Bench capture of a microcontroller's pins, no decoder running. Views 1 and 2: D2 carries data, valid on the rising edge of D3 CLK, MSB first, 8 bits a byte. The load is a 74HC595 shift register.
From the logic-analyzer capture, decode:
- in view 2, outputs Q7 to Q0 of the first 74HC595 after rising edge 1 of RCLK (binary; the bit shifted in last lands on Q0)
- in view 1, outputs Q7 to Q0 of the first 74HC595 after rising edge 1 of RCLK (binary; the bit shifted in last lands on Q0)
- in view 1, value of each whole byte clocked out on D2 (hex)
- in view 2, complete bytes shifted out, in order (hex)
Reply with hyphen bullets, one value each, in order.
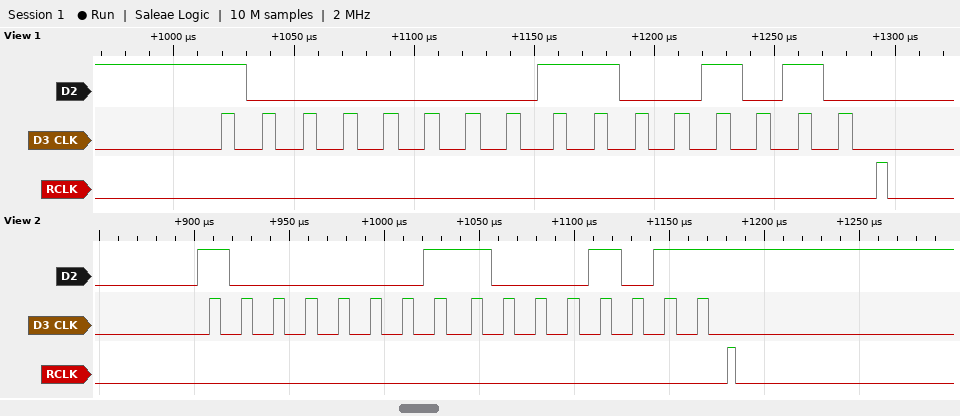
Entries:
- 10001011
- 11001010
- 80 CA
- 0x81 0x8B
